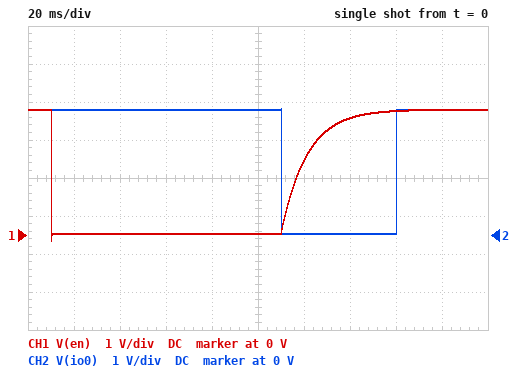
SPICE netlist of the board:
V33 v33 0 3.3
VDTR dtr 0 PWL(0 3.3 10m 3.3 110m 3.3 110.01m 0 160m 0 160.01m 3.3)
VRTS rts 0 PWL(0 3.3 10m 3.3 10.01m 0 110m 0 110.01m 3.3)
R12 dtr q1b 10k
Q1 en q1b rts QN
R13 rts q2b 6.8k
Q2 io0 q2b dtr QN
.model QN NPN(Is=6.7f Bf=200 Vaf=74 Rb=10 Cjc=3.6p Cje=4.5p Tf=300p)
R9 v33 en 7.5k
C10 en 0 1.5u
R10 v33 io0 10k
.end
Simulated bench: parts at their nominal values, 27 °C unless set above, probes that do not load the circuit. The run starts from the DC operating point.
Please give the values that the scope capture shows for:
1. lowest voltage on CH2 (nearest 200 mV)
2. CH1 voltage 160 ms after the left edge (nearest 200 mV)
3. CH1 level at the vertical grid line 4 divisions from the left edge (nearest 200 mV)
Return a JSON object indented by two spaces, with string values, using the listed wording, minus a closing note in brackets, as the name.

{
  "lowest voltage on CH2": "0 V",
  "CH1 voltage 160 ms after the left edge": "3.2 V",
  "CH1 level at the vertical grid line 4 divisions from the left edge": "0 V"
}
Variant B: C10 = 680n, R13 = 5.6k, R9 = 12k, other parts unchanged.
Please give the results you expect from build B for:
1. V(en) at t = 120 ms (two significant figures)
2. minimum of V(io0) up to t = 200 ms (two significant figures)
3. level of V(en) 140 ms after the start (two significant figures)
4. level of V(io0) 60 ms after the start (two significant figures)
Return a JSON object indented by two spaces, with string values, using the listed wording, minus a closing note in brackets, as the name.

{
  "V(en) at t = 120 ms": "2.3 V",
  "minimum of V(io0) up to t = 200 ms": "26 mV",
  "level of V(en) 140 ms after the start": "3.2 V",
  "level of V(io0) 60 ms after the start": "3.3 V"
}
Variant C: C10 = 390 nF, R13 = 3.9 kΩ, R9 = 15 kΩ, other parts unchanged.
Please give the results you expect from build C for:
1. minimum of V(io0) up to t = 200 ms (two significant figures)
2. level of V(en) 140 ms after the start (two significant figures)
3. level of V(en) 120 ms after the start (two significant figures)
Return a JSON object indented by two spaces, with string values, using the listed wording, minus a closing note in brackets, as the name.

{
  "minimum of V(io0) up to t = 200 ms": "24 mV",
  "level of V(en) 140 ms after the start": "3.3 V",
  "level of V(en) 120 ms after the start": "2.7 V"
}
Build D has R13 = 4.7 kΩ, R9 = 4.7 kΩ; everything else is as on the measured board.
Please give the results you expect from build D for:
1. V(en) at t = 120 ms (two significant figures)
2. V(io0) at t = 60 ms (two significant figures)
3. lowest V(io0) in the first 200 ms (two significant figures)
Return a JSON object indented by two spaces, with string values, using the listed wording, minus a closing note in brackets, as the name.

{
  "V(en) at t = 120 ms": "2.5 V",
  "V(io0) at t = 60 ms": "3.3 V",
  "lowest V(io0) in the first 200 ms": "25 mV"
}
